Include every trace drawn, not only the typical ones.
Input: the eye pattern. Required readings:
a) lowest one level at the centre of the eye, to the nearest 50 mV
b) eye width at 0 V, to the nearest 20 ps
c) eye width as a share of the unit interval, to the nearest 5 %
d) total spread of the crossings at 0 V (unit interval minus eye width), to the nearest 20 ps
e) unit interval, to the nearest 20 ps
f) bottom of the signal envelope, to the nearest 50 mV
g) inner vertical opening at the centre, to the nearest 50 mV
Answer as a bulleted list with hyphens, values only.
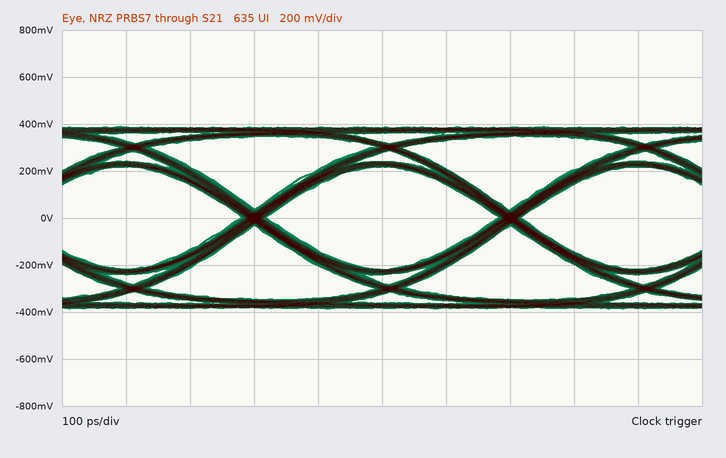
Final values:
- 200 mV
- 360 ps
- 90 %
- 40 ps
- 400 ps
- -400 mV
- 450 mV
